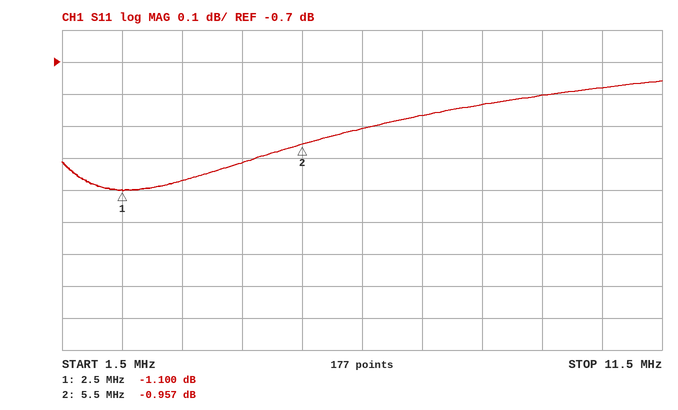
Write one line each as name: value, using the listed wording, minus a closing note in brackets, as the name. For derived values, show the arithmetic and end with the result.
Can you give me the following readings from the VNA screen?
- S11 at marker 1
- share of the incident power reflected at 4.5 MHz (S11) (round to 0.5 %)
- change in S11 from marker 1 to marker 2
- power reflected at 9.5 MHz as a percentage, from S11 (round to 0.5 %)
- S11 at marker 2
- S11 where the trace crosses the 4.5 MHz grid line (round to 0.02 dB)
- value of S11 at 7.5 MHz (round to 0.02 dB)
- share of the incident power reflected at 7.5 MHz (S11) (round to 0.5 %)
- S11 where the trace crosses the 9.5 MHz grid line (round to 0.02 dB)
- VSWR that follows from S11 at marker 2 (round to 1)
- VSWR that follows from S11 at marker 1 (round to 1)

S11 at marker 1: -1.100 dB
share of the incident power reflected at 4.5 MHz (S11): 10^(-1.02/10) ≈ 79.1 %, so 79.0 % to the nearest 0.5 %
change in S11 from marker 1 to marker 2: -0.957 − (-1.1) = 0.143 dB
power reflected at 9.5 MHz as a percentage, from S11: 10^(-0.8/10) ≈ 83.2 %, so 83.0 % to the nearest 0.5 %
S11 at marker 2: -0.957 dB
S11 where the trace crosses the 4.5 MHz grid line: -1.02 dB
value of S11 at 7.5 MHz: -0.86 dB
share of the incident power reflected at 7.5 MHz (S11): 10^(-0.86/10) ≈ 82.0 %
S11 where the trace crosses the 9.5 MHz grid line: -0.80 dB
VSWR that follows from S11 at marker 2: (1 + 0.8957)/(1 − 0.8957) ≈ 18
VSWR that follows from S11 at marker 1: (1 + 0.8810)/(1 − 0.8810) ≈ 16
